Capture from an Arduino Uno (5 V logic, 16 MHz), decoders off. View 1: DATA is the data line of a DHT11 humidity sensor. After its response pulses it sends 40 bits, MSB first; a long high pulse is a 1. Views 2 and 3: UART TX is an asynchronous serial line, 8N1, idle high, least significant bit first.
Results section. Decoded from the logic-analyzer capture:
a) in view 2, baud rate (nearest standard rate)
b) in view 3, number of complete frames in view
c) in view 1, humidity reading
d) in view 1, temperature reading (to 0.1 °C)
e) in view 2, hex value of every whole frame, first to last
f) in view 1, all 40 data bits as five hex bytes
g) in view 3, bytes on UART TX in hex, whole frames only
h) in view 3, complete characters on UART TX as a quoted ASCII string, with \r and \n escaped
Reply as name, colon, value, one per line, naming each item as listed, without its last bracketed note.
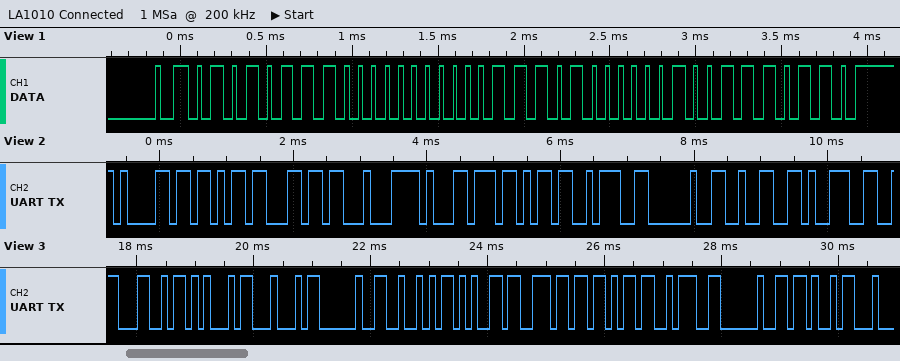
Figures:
in view 2, baud rate: 9600 baud
in view 3, number of complete frames in view: 11
in view 1, humidity reading: 87 %
in view 1, temperature reading: 29.2 °C
in view 2, hex value of every whole frame, first to last: 0x61 0x6B 0x6C 0xC4 0xB1 0x6B 0x3A 0x20 0x32 0x39
in view 1, all 40 data bits as five hex bytes: 57 00 1D 02 76
in view 3, bytes on UART TX in hex, whole frames only: 4C 45 44 20 52 65 6E 6B 3A 20 4B
in view 3, complete characters on UART TX as a quoted ASCII string, with \r and \n escaped: "LED Renk: K"
